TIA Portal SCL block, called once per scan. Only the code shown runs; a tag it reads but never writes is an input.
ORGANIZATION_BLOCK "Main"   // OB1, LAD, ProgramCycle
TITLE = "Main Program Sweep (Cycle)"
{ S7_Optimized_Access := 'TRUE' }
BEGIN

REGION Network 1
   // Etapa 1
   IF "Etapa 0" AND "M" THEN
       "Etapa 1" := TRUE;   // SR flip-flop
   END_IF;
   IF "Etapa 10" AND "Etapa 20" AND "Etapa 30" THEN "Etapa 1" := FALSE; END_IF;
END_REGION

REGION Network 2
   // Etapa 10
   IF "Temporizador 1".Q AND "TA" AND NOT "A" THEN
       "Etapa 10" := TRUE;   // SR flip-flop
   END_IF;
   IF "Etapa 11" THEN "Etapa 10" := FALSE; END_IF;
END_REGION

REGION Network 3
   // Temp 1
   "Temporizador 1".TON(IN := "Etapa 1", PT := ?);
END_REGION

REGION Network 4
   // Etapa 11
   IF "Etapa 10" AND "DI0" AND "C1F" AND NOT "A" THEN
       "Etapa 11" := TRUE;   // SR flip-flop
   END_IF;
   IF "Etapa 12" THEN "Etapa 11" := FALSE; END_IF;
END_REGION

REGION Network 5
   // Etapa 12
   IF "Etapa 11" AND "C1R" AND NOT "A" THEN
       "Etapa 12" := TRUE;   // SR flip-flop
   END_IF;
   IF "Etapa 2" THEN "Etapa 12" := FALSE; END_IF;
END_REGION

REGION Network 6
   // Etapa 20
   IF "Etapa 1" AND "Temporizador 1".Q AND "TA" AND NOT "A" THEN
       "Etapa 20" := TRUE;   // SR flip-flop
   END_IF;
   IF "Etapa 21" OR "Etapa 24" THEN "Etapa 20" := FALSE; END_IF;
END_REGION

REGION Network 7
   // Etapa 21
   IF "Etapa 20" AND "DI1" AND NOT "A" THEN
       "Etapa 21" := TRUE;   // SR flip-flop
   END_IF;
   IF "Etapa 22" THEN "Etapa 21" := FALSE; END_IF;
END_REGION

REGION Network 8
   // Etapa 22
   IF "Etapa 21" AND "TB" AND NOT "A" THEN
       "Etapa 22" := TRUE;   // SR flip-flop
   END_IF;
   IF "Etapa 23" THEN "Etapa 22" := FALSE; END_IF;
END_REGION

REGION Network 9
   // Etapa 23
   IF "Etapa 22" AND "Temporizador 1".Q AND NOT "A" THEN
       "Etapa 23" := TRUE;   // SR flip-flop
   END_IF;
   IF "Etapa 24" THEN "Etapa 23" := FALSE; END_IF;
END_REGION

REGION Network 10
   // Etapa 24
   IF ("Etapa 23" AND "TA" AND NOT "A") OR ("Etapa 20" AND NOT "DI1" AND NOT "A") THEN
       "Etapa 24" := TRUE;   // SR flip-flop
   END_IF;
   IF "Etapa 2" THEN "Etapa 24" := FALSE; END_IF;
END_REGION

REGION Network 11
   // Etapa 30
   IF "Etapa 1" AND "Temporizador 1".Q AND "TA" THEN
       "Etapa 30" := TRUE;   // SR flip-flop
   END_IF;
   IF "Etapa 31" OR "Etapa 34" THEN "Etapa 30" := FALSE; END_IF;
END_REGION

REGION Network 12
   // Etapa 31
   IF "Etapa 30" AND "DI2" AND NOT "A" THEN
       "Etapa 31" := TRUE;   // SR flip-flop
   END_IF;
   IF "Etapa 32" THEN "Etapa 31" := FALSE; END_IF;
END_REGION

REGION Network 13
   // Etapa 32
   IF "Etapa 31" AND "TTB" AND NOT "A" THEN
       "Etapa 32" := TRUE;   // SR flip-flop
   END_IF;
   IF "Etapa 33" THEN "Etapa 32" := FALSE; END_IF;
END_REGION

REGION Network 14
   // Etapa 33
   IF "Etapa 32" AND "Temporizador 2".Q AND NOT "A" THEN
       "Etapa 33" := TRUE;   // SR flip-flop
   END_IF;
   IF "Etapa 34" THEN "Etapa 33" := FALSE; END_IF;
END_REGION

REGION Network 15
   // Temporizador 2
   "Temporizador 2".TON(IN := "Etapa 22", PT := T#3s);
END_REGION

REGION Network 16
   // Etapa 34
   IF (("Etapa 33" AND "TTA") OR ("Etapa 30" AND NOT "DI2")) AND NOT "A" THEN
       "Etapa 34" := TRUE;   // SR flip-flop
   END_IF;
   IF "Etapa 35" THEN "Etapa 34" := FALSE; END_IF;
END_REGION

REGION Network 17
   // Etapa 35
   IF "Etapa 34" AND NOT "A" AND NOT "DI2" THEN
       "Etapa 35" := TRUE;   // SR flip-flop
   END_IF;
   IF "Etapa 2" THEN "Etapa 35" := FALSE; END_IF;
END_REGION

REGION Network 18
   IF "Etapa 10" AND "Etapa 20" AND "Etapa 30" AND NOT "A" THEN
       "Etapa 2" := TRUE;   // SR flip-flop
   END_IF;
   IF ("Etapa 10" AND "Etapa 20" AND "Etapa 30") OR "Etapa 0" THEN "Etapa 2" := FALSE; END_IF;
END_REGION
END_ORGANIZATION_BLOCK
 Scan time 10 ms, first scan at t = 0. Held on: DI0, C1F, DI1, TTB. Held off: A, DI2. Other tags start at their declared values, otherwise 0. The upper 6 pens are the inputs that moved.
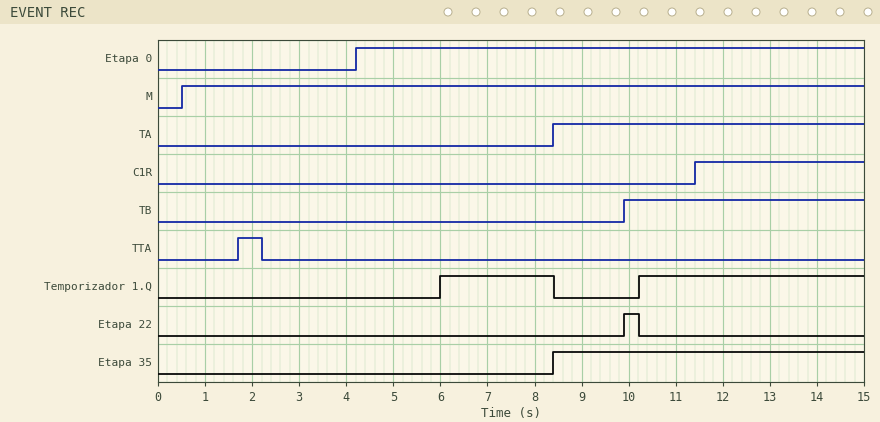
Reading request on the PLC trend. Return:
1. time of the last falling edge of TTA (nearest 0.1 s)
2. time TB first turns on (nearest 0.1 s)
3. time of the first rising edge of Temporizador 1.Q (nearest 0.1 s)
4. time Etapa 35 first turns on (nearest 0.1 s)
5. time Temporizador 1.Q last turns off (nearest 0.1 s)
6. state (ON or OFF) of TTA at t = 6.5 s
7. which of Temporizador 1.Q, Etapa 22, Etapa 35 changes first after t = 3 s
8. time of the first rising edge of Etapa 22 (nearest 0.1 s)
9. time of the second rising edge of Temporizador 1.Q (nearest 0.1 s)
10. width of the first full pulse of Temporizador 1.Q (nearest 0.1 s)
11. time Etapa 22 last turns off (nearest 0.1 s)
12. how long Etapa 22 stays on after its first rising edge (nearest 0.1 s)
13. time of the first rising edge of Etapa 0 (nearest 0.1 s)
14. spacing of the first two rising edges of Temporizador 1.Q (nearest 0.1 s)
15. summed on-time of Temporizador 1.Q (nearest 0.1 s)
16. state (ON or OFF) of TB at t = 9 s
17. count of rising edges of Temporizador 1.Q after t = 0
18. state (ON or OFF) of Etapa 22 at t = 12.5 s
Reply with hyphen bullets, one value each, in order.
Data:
- 2.2 s
- 9.9 s
- 6.0 s
- 8.4 s
- 8.4 s
- OFF
- Temporizador 1.Q
- 9.9 s
- 10.2 s
- 2.4 s
- 10.2 s
- 0.3 s
- 4.2 s
- 4.2 s
- 7.2 s
- OFF
- 2
- OFF
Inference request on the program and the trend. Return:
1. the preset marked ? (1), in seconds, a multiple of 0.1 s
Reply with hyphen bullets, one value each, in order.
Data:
- 1.8 s
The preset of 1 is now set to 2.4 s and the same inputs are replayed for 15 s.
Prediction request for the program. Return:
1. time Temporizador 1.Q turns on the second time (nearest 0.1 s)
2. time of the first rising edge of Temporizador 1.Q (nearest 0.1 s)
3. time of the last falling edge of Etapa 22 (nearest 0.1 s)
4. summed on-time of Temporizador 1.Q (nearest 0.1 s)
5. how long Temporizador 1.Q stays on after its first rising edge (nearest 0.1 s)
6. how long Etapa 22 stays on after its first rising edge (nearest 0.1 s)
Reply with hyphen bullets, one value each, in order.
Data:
- 10.8 s
- 6.6 s
- 10.8 s
- 6.0 s
- 1.8 s
- 0.9 s
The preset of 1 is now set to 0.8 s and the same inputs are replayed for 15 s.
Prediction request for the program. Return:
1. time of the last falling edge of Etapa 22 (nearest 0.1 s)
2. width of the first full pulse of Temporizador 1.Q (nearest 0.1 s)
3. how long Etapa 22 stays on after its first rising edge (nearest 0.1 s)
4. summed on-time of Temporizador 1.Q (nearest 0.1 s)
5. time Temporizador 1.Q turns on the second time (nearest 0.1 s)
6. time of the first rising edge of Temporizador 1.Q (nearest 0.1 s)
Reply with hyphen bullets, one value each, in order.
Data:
- 9.9 s
- 3.4 s
- 0.0 s
- 9.2 s
- 9.2 s
- 5.0 s
